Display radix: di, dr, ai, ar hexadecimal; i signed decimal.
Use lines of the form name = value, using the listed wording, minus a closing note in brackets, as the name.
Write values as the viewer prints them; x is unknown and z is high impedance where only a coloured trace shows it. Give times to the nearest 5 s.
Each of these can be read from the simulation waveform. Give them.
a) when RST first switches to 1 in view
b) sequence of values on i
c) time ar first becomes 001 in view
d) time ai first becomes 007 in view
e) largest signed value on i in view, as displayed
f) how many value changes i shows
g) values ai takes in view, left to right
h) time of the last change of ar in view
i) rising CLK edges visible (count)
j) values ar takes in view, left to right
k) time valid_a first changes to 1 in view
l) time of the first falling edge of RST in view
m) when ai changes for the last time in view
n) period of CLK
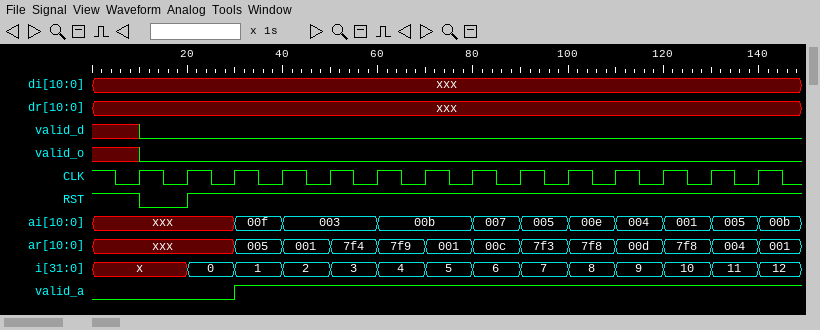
when RST first switches to 1 in view = 20 s
sequence of values on i = x, 0, 1, 2, 3, 4, 5, 6, 7, 8, 9, 10, 11, 12
time ar first becomes 001 in view = 40 s
time ai first becomes 007 in view = 80 s
largest signed value on i in view, as displayed = 12
how many value changes i shows = 13
values ai takes in view, left to right = xxx, 00f, 003, 00b, 007, 005, 00e, 004, 001, 005, 00b
time of the last change of ar in view = 140 s
rising CLK edges visible = 14
values ar takes in view, left to right = xxx, 005, 001, 7f4, 7f9, 001, 00c, 7f3, 7f8, 00d, 7f8, 004, 001
time valid_a first changes to 1 in view = 30 s
time of the first falling edge of RST in view = 10 s
when ai changes for the last time in view = 140 s
period of CLK = 10 s
